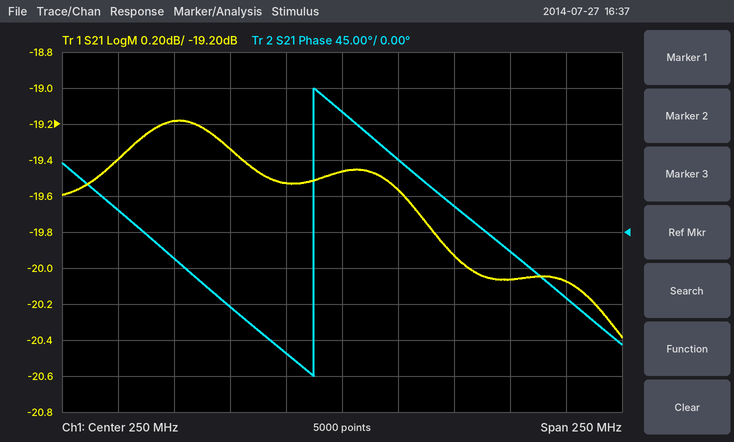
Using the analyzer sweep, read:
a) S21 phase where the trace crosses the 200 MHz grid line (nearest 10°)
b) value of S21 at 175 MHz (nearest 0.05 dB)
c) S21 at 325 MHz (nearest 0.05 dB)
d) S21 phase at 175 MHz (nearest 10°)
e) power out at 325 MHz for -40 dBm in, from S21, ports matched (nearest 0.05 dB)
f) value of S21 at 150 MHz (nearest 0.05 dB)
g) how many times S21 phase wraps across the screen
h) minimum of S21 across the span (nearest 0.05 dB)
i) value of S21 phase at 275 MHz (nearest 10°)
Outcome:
-90°
-19.20 dB
-20.05 dB
-30°
-60.05 dBm
-19.40 dB
1
-20.40 dB
90°
